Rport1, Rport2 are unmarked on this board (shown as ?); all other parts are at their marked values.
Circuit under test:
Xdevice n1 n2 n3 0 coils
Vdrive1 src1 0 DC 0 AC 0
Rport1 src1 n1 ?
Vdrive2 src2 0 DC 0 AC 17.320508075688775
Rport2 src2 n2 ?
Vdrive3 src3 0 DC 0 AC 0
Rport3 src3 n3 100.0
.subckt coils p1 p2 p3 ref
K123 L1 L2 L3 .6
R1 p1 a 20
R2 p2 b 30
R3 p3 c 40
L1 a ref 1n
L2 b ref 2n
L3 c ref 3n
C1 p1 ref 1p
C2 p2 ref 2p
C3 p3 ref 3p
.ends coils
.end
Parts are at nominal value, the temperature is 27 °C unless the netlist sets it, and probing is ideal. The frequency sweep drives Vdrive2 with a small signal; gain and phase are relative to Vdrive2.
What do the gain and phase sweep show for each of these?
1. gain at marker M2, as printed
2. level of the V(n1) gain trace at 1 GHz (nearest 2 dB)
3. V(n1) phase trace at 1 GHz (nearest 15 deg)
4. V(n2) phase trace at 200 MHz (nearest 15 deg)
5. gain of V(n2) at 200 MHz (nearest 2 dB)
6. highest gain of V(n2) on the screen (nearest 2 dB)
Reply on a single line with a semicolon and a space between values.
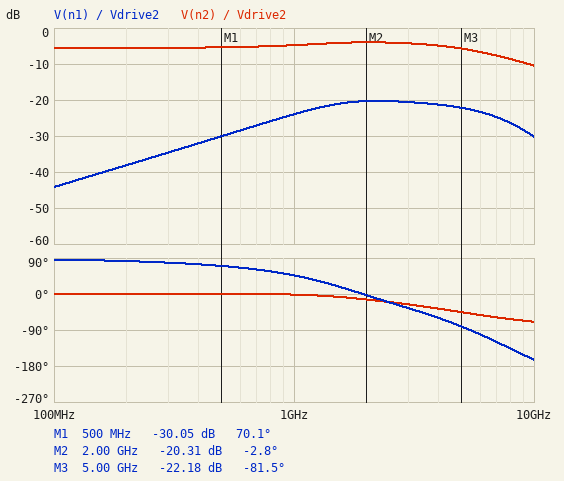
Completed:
-20.31 dB; -24 dB; 45 deg; 0 deg; -6 dB; -4 dB
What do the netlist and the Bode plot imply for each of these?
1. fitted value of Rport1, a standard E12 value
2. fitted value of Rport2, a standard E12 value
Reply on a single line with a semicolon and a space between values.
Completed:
39 Ω; 27 Ω
